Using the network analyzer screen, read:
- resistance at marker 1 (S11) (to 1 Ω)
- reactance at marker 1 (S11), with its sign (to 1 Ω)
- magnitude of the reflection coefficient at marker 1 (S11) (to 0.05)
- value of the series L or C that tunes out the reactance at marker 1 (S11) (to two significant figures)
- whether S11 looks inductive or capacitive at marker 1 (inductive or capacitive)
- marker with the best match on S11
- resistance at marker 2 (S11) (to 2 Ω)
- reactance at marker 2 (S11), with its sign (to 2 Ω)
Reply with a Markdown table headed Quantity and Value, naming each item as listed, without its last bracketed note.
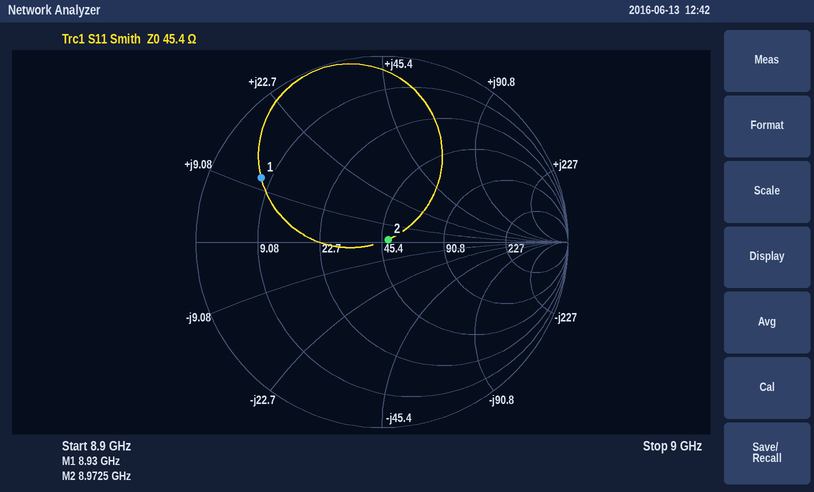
| Quantity | Value |
|---|---|
| resistance at marker 1 (S11) | 7 Ω |
| reactance at marker 1 (S11), with its sign | +11 Ω |
| magnitude of the reflection coefficient at marker 1 (S11) | 0.75 |
| value of the series L or C that tunes out the reactance at marker 1 (S11) | 1.6 pF |
| whether S11 looks inductive or capacitive at marker 1 | inductive |
| marker with the best match on S11 | marker 2 |
| resistance at marker 2 (S11) | 48 Ω |
| reactance at marker 2 (S11), with its sign | +2 Ω |
